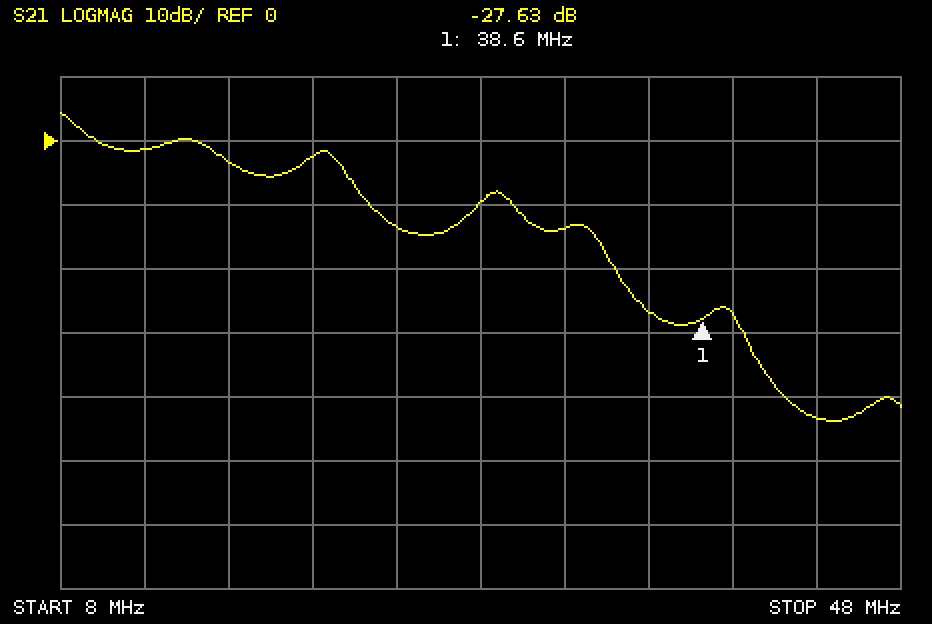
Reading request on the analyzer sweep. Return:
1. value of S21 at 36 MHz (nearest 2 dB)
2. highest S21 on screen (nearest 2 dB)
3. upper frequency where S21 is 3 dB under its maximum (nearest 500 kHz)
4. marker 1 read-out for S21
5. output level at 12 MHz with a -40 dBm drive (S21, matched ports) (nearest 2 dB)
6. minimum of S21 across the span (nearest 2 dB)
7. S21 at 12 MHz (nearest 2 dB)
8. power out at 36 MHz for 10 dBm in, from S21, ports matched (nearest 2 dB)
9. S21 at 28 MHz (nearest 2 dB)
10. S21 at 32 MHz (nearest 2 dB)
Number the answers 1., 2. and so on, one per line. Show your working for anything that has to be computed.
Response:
1. -26 dB
2. 4 dB
3. 9.0 MHz
4. -27.63 dB
5. -40 dBm + (-2 dB) = -42 dBm
6. -44 dB
7. -2 dB
8. 10 dBm + (-26 dB) = -16 dBm
9. -10 dB
10. -14 dB
